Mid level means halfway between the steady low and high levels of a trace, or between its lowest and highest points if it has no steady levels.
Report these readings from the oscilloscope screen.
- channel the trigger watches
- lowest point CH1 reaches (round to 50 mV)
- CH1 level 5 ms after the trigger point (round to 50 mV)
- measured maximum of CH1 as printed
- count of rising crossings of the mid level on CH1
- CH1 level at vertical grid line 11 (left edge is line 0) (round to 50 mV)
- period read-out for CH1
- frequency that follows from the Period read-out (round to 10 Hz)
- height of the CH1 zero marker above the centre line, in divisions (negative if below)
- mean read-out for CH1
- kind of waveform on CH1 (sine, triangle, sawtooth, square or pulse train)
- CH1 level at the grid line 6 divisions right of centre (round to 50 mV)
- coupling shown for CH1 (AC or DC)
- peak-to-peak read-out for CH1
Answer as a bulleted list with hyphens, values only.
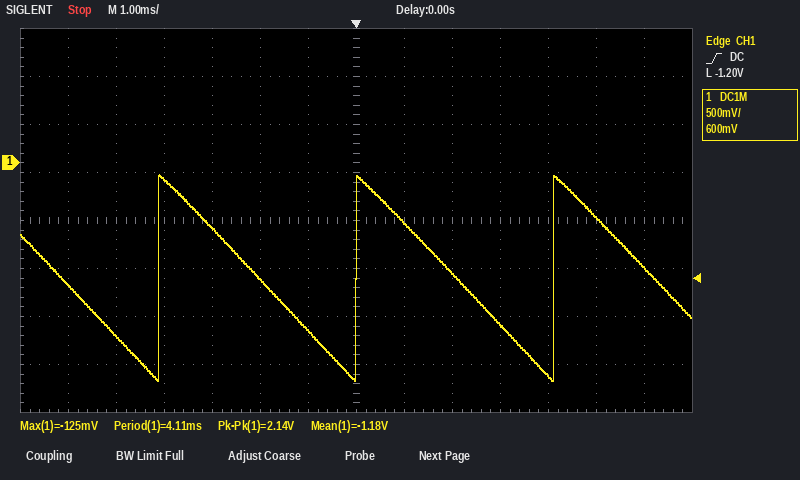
- CH1
- -2.25 V
- -550 mV
- -125 mV
- 3
- -2.20 V
- 4.11 ms
- 240 Hz
- +1.2 div
- -1.18 V
- sawtooth
- -1.10 V
- DC
- 2.14 V
